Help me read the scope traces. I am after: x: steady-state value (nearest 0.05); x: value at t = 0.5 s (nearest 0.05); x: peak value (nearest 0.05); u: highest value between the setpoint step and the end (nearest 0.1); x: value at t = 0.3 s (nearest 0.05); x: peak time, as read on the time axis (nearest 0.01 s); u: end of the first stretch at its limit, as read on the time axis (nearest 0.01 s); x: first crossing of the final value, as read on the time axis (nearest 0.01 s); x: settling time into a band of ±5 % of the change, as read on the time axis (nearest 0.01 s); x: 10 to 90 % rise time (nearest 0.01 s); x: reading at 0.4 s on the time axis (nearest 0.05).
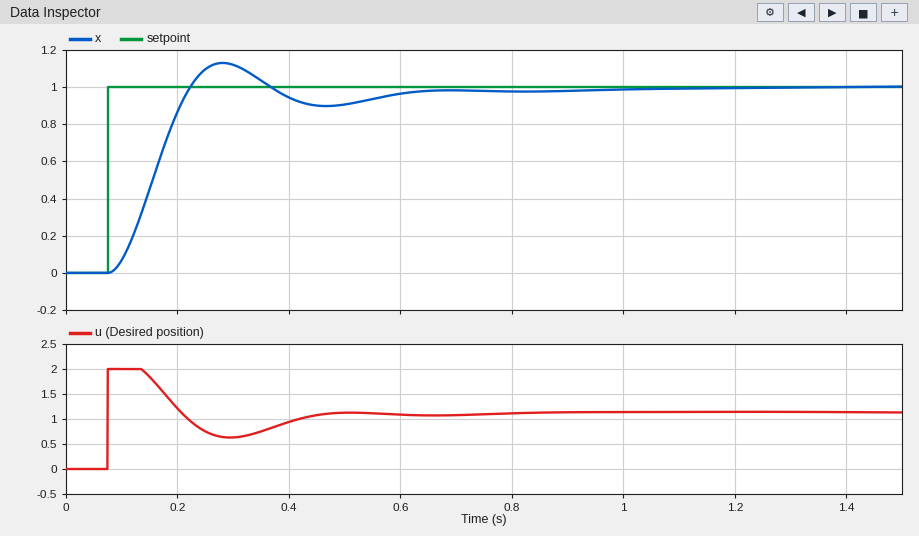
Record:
1.00
0.90
1.15
2.0
1.10
0.28 s
0.14 s
0.22 s
0.57 s
0.10 s
0.95
